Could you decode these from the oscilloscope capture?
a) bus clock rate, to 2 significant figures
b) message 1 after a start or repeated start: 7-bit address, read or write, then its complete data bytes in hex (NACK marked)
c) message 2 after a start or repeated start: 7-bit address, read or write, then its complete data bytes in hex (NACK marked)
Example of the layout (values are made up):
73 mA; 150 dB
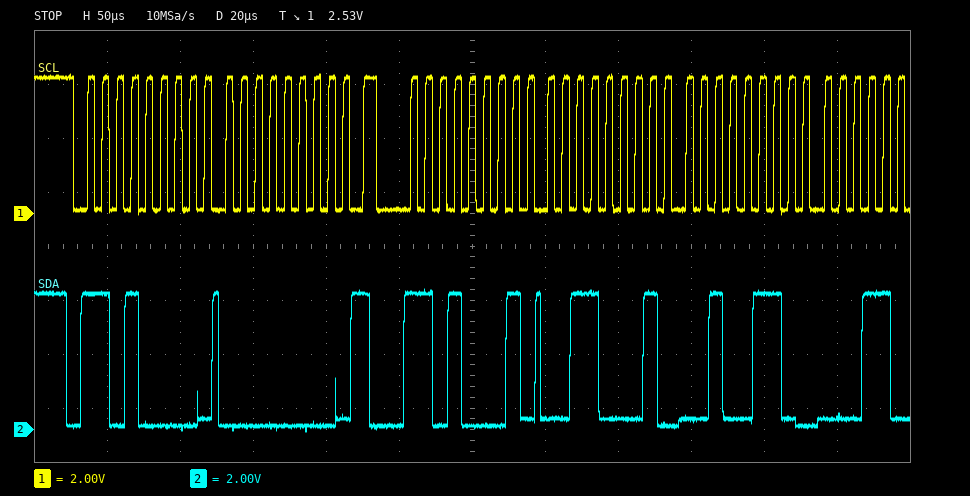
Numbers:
100 kHz; 0x68 write: 00; 0x68 read: 31 26
